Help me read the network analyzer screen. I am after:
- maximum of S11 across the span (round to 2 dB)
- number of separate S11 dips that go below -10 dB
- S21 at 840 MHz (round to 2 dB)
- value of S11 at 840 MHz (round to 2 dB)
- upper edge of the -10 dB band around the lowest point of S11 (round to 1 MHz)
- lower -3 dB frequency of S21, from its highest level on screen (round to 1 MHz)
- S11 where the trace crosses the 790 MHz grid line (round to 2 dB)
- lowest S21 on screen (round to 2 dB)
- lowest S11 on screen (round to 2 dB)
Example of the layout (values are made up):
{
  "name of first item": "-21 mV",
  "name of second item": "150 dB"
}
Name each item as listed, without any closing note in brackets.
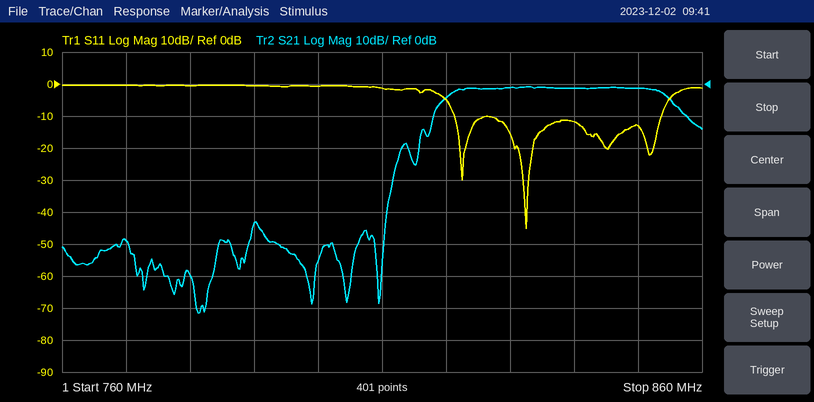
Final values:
{
  "maximum of S11 across the span": "0 dB",
  "number of separate S11 dips that go below -10 dB": "4",
  "S21 at 840 MHz": "-2 dB",
  "value of S11 at 840 MHz": "-12 dB",
  "upper edge of the -10 dB band around the lowest point of S11": "854 MHz",
  "lower -3 dB frequency of S21, from its highest level on screen": "820 MHz",
  "S11 where the trace crosses the 790 MHz grid line": "0 dB",
  "lowest S21 on screen": "-72 dB",
  "lowest S11 on screen": "-46 dB"
}
